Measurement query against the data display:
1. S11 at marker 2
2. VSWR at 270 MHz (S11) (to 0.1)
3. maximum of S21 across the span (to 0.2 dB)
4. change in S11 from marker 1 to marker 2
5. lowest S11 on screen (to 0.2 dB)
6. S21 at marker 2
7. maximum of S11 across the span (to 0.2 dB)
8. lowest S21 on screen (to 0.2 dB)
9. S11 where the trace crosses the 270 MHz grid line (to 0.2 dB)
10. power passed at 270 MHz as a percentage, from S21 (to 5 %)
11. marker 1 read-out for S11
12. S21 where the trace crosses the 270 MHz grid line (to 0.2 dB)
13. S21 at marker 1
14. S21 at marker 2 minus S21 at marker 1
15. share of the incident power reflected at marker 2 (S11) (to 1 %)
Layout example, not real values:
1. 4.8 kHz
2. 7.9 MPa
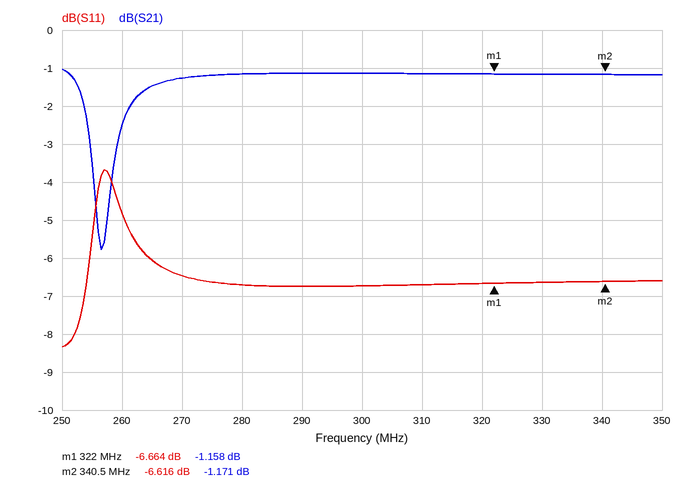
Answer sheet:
1. -6.616 dB
2. 2.8
3. -1.0 dB
4. 0.048 dB
5. -8.4 dB
6. -1.171 dB
7. -3.6 dB
8. -5.8 dB
9. -6.4 dB
10. 75 %
11. -6.664 dB
12. -1.2 dB
13. -1.158 dB
14. -0.013 dB
15. 22 %
